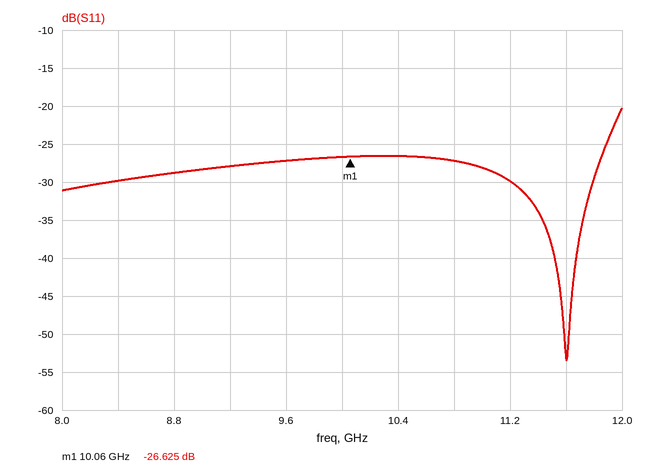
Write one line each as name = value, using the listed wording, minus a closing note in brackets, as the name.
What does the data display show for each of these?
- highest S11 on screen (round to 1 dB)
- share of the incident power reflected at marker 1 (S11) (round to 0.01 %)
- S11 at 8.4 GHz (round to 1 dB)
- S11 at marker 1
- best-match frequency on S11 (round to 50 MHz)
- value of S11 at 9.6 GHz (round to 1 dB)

highest S11 on screen = -20 dB
share of the incident power reflected at marker 1 (S11) = 0.22 %
S11 at 8.4 GHz = -30 dB
S11 at marker 1 = -26.625 dB
best-match frequency on S11 = 11.60 GHz
value of S11 at 9.6 GHz = -27 dB
